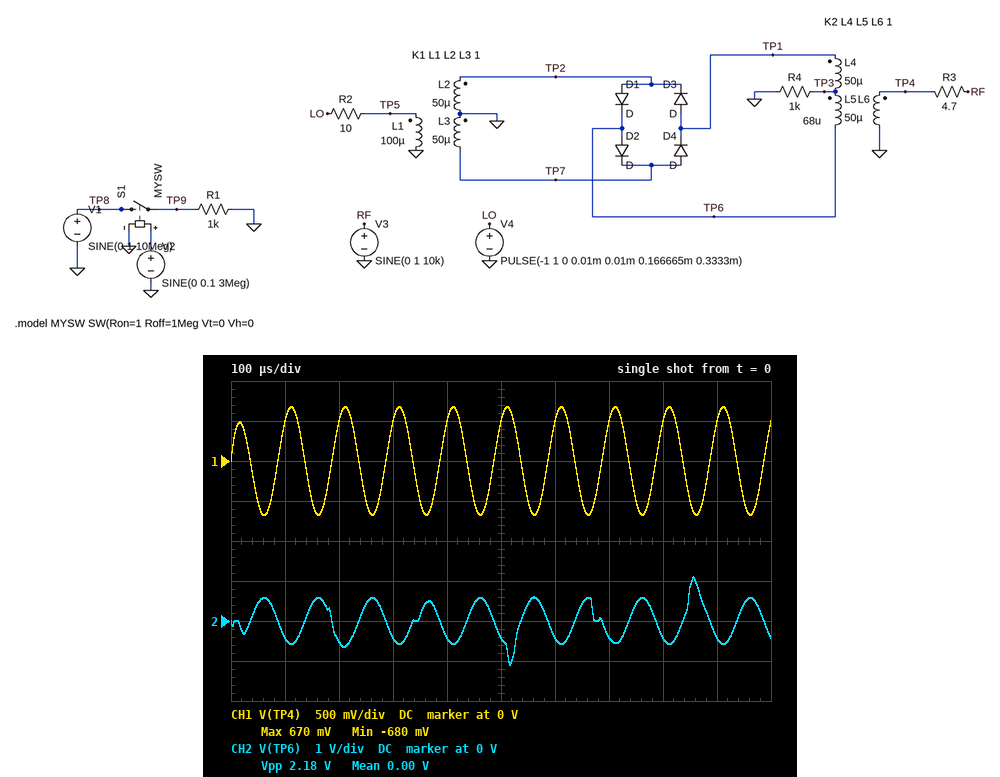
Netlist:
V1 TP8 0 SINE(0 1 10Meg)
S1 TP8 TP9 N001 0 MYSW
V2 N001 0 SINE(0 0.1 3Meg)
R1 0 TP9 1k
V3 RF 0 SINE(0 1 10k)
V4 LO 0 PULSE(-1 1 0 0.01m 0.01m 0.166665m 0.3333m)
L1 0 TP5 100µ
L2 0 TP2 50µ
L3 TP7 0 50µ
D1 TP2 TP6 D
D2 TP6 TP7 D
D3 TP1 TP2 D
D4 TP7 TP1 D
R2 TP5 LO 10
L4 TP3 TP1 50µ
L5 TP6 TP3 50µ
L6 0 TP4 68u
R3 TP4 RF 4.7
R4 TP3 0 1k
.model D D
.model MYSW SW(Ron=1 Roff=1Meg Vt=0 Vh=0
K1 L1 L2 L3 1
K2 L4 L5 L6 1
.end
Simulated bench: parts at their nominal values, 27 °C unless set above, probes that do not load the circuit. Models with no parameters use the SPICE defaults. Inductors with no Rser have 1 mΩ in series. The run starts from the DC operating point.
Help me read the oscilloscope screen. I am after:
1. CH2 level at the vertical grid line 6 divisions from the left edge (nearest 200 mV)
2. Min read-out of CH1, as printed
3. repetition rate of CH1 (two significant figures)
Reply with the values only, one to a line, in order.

-400 mV
-680 mV
10 kHz
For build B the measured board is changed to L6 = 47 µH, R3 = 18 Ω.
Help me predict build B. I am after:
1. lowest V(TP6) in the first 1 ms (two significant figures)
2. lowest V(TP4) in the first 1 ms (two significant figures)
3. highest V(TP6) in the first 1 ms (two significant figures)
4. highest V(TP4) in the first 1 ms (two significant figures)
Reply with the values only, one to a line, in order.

-240 mV
-160 mV
330 mV
160 mV
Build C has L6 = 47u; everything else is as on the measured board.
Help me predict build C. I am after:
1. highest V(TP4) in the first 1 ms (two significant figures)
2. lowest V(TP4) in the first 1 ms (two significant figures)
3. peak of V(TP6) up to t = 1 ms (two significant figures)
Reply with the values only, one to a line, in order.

530 mV
-530 mV
1.1 V
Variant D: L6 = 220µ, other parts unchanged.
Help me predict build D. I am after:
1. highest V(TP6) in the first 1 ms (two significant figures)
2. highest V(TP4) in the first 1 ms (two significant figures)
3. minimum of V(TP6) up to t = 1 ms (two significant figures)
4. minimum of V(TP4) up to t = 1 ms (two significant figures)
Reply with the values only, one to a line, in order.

640 mV
950 mV
-900 mV
-1.0 V
